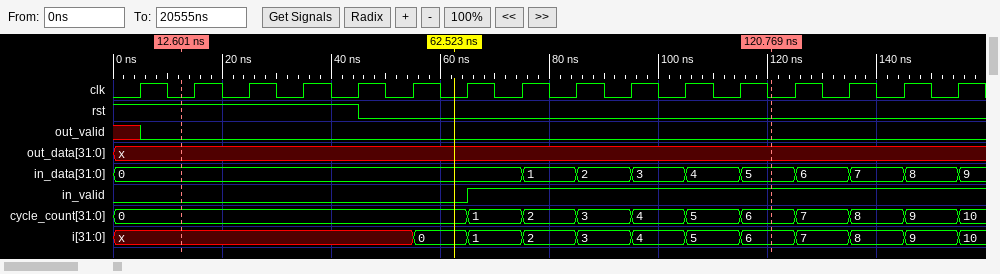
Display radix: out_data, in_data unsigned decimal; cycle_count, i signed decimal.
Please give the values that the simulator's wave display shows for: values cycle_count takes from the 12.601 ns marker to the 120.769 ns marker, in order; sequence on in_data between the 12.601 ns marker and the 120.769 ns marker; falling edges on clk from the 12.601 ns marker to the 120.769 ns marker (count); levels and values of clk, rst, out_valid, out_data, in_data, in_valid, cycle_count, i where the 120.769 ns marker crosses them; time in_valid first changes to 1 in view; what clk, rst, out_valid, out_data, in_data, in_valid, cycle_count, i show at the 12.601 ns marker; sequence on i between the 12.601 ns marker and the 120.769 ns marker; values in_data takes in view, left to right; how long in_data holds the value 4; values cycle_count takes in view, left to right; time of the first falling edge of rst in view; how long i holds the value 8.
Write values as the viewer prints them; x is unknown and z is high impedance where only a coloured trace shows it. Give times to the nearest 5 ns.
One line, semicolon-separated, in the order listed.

0, 1, 2, 3, 4, 5, 6; 0, 1, 2, 3, 4, 5; 11; clk=0, rst=0, out_valid=0, out_data=x, in_data=5, in_valid=1, cycle_count=6, i=6; 65 ns; clk=0, rst=1, out_valid=0, out_data=x, in_data=0, in_valid=0, cycle_count=0, i=x; x, 0, 1, 2, 3, 4, 5, 6; 0, 1, 2, 3, 4, 5, 6, 7, 8, 9; 10 ns; 0, 1, 2, 3, 4, 5, 6, 7, 8, 9, 10; 45 ns; 10 ns
